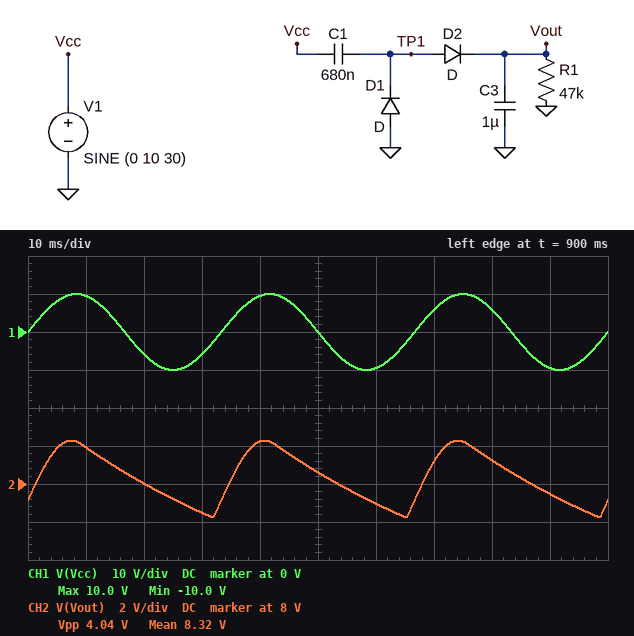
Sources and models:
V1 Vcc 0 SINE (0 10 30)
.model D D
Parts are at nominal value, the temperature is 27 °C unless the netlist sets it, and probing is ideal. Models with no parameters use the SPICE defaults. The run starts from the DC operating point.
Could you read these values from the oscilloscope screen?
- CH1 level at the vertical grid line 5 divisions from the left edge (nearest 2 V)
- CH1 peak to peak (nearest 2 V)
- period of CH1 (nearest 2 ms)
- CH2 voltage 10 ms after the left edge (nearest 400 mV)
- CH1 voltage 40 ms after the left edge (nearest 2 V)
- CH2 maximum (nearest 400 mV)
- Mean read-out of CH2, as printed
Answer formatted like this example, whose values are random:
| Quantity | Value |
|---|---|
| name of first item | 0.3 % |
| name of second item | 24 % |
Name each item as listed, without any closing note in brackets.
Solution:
| Quantity | Value |
|---|---|
| CH1 level at the vertical grid line 5 divisions from the left edge | 0 V |
| CH1 peak to peak | 20 V |
| period of CH1 | 34 ms |
| CH2 voltage 10 ms after the left edge | 10.0 V |
| CH1 voltage 40 ms after the left edge | 10 V |
| CH2 maximum | 10.4 V |
| Mean read-out of CH2, as printed | 8.32 V |
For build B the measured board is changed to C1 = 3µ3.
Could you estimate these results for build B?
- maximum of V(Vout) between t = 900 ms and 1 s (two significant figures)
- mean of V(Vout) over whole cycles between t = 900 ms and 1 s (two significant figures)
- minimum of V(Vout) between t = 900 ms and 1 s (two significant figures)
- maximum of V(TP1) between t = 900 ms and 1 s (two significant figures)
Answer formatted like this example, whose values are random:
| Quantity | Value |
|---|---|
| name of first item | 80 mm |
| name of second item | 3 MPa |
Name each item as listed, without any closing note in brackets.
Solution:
| Quantity | Value |
|---|---|
| maximum of V(Vout) between t = 900 ms and 1 s | 16 V |
| mean of V(Vout) over whole cycles between t = 900 ms and 1 s | 13 V |
| minimum of V(Vout) between t = 900 ms and 1 s | 9.5 V |
| maximum of V(TP1) between t = 900 ms and 1 s | 17 V |
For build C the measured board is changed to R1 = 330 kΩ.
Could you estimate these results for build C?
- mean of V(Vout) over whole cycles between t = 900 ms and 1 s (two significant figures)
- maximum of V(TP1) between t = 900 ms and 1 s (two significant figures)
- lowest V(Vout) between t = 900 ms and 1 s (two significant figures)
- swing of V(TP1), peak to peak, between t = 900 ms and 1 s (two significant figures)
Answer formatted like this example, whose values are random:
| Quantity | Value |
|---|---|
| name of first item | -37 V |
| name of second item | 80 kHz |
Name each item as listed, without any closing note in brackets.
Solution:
| Quantity | Value |
|---|---|
| mean of V(Vout) over whole cycles between t = 900 ms and 1 s | 16 V |
| maximum of V(TP1) between t = 900 ms and 1 s | 17 V |
| lowest V(Vout) between t = 900 ms and 1 s | 15 V |
| swing of V(TP1), peak to peak, between t = 900 ms and 1 s | 18 V |
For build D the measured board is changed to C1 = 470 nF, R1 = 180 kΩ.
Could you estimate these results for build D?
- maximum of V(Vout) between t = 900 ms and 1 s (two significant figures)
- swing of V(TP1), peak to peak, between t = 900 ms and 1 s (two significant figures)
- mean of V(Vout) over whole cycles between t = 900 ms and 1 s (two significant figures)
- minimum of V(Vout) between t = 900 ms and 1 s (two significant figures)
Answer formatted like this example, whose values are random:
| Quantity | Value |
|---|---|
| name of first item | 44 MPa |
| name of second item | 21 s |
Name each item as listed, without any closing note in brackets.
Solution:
| Quantity | Value |
|---|---|
| maximum of V(Vout) between t = 900 ms and 1 s | 14 V |
| swing of V(TP1), peak to peak, between t = 900 ms and 1 s | 15 V |
| mean of V(Vout) over whole cycles between t = 900 ms and 1 s | 13 V |
| minimum of V(Vout) between t = 900 ms and 1 s | 12 V |
